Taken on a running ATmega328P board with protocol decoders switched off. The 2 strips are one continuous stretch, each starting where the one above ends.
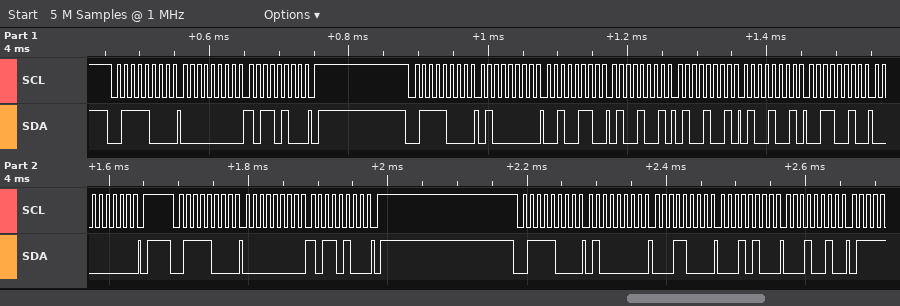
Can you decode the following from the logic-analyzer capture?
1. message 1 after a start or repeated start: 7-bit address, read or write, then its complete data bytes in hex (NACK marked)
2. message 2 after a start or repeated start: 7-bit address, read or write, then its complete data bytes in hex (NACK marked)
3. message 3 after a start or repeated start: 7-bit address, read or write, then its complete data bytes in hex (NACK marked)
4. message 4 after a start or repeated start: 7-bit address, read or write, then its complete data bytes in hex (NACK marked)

0x3C write: 00 B4
0x3C write: 40 26 49 49 49 32 00
0x3C write: 00 B4
0x3C write: 40 18 14 12
